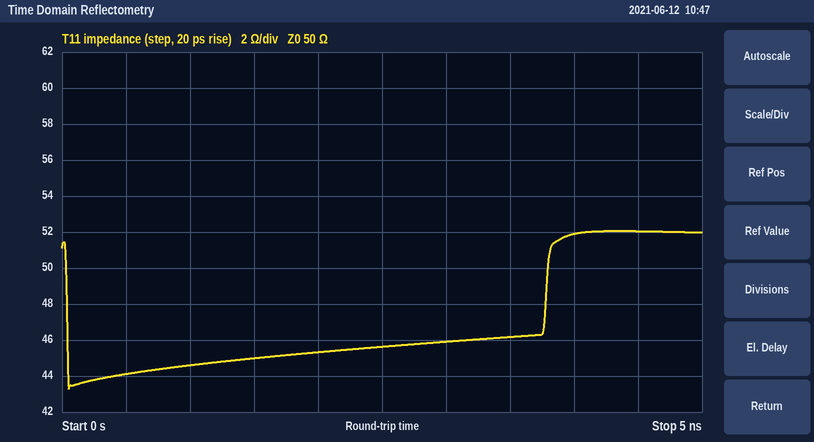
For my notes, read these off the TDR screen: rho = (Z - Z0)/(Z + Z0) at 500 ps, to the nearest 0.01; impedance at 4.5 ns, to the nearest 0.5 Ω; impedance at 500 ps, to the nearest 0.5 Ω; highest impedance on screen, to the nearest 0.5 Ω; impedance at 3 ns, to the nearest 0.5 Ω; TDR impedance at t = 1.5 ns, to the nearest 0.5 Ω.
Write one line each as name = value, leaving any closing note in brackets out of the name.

rho = (Z - Z0)/(Z + Z0) at 500 ps, to the nearest 0.01 = -0.06
impedance at 4.5 ns, to the nearest 0.5 Ω = 52.0 Ω
impedance at 500 ps, to the nearest 0.5 Ω = 44.0 Ω
highest impedance on screen, to the nearest 0.5 Ω = 52.0 Ω
impedance at 3 ns, to the nearest 0.5 Ω = 46.0 Ω
TDR impedance at t = 1.5 ns, to the nearest 0.5 Ω = 45.0 Ω
